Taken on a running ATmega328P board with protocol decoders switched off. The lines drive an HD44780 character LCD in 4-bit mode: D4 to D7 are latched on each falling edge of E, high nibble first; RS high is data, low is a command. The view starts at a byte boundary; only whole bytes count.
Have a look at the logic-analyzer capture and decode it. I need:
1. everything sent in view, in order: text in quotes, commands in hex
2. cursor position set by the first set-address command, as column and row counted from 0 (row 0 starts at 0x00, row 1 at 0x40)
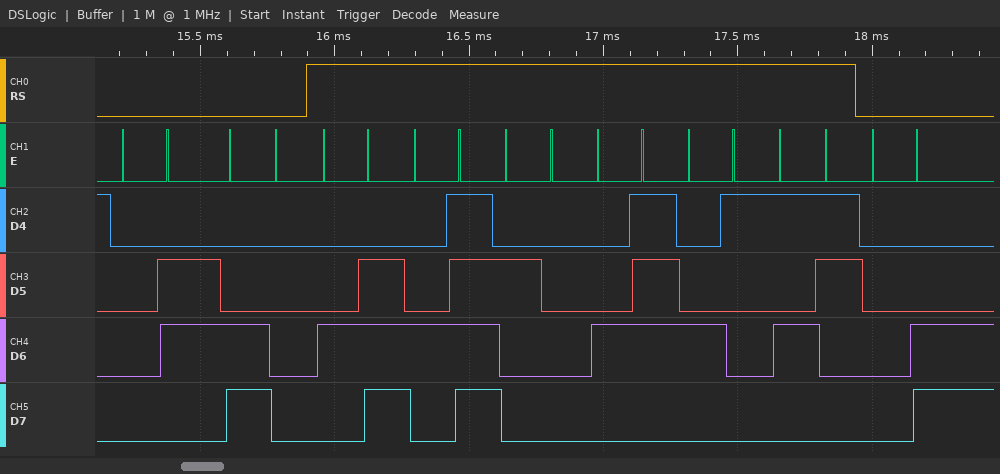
0x06 0xC0 "NO GAS" 0x0C
column 0, row 1
